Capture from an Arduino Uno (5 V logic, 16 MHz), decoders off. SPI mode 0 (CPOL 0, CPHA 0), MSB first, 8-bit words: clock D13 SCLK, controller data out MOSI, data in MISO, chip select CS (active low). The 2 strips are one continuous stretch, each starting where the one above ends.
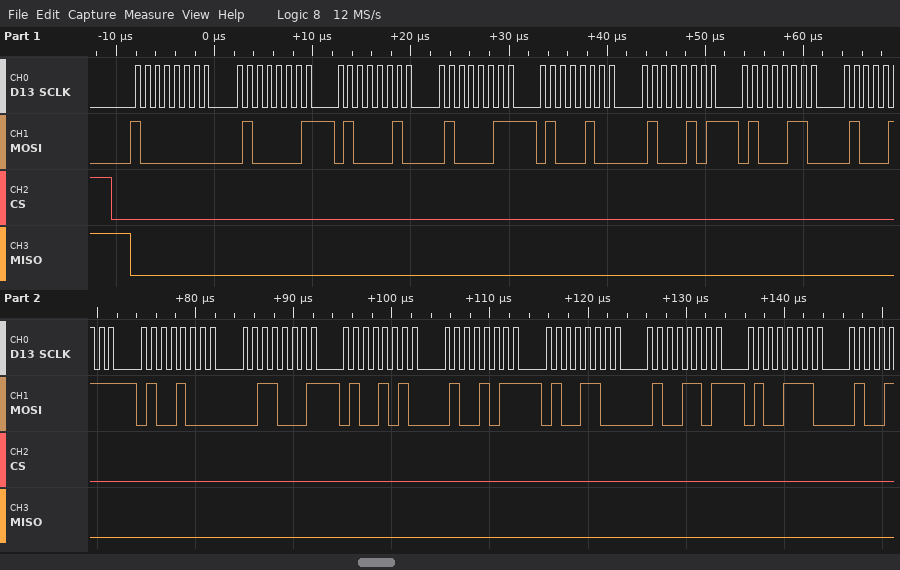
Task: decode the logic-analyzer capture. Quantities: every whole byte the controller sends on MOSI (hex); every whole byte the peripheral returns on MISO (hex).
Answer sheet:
0x80 0x41 0x42 0x43 0x44 0x45 0x46 0x47 0x48 0x31 0x4A 0x4B 0x4C 0x4D 0x4E
0x00 0x00 0x00 0x00 0x00 0x00 0x00 0x00 0x00 0x00 0x00 0x00 0x00 0x00 0x00
